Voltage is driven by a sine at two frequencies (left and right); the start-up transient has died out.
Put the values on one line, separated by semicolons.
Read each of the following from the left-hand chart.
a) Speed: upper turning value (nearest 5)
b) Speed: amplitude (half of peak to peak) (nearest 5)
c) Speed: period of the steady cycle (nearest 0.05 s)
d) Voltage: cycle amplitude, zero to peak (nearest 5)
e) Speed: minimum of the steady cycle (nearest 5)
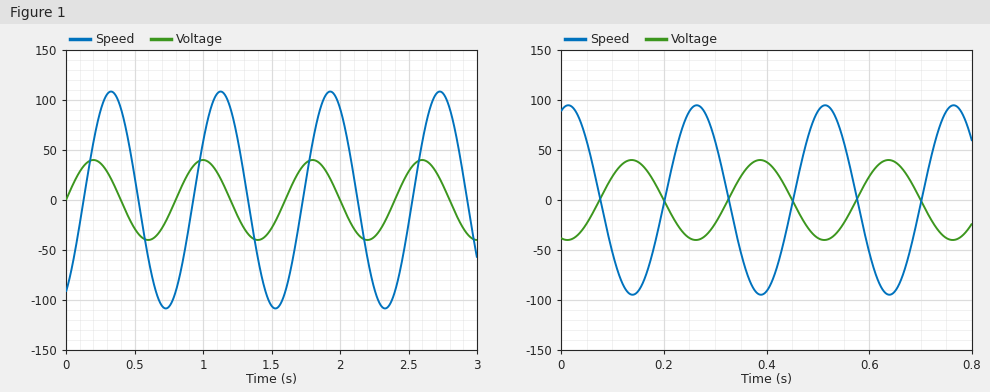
110; 110; 0.80 s; 40; -110
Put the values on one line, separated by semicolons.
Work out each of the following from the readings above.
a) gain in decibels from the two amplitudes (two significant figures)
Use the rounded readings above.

8.8 dB
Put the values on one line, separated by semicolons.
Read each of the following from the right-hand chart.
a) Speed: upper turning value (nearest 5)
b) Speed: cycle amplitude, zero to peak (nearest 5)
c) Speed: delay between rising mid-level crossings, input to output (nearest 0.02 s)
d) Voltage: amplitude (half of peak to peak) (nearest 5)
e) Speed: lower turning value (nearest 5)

95; 95; 0.12 s; 40; -95
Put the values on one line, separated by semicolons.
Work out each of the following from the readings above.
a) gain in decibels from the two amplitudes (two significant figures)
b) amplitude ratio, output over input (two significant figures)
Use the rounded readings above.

7.5 dB; 2.4
